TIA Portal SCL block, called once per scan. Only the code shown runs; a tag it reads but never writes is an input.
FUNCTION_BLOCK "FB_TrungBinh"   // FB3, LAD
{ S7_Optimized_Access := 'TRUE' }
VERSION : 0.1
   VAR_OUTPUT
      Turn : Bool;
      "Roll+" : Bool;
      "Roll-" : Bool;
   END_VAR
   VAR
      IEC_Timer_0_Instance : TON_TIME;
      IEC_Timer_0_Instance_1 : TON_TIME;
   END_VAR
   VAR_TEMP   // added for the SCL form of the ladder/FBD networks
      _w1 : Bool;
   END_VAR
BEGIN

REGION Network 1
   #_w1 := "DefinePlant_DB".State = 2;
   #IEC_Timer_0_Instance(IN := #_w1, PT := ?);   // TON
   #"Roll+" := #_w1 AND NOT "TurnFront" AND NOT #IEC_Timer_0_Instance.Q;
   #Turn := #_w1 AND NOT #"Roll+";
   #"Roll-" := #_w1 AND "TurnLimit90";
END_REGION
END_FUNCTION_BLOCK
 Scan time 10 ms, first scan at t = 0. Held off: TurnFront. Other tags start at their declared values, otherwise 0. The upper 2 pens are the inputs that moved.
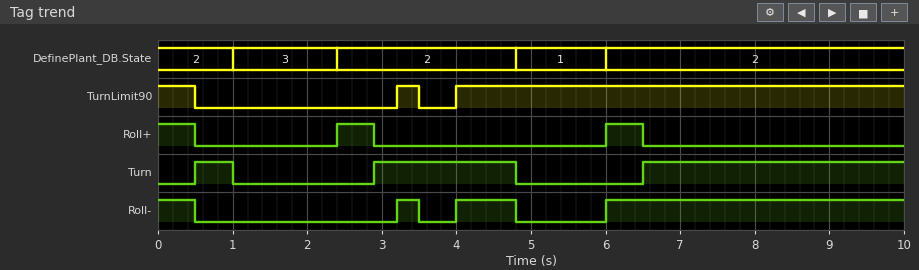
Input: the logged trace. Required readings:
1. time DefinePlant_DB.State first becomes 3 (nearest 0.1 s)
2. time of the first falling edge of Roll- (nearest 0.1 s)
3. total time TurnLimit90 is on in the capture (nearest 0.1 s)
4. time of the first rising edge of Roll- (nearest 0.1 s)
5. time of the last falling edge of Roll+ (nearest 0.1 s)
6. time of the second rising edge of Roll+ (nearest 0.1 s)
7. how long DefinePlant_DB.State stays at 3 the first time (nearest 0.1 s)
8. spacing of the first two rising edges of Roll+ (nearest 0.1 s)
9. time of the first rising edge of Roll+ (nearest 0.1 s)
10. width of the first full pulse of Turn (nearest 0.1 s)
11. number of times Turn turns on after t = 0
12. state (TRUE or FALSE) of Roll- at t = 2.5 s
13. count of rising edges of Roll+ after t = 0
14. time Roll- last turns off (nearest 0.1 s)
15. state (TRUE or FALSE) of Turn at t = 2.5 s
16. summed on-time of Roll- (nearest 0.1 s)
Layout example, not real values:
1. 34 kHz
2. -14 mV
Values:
1. 1.0 s
2. 0.5 s
3. 6.8 s
4. 3.2 s
5. 6.5 s
6. 6.0 s
7. 1.4 s
8. 3.6 s
9. 2.4 s
10. 0.5 s
11. 3
12. FALSE
13. 2
14. 4.8 s
15. FALSE
16. 5.6 s
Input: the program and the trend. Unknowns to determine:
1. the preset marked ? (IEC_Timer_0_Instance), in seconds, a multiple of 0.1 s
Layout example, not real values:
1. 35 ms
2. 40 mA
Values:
1. 0.5 s
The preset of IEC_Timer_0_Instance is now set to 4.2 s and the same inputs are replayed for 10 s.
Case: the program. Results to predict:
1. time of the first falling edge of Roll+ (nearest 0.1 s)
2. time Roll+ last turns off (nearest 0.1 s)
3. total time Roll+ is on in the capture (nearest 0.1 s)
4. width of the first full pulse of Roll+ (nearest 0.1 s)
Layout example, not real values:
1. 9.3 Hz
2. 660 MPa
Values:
1. 1.0 s
2. 4.8 s
3. 7.4 s
4. 2.4 s
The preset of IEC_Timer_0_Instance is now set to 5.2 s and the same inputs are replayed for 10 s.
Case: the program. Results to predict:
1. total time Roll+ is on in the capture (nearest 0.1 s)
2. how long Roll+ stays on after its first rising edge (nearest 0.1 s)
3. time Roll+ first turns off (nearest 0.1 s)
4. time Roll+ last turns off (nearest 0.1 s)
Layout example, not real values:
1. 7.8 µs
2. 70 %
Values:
1. 7.4 s
2. 2.4 s
3. 1.0 s
4. 4.8 s
